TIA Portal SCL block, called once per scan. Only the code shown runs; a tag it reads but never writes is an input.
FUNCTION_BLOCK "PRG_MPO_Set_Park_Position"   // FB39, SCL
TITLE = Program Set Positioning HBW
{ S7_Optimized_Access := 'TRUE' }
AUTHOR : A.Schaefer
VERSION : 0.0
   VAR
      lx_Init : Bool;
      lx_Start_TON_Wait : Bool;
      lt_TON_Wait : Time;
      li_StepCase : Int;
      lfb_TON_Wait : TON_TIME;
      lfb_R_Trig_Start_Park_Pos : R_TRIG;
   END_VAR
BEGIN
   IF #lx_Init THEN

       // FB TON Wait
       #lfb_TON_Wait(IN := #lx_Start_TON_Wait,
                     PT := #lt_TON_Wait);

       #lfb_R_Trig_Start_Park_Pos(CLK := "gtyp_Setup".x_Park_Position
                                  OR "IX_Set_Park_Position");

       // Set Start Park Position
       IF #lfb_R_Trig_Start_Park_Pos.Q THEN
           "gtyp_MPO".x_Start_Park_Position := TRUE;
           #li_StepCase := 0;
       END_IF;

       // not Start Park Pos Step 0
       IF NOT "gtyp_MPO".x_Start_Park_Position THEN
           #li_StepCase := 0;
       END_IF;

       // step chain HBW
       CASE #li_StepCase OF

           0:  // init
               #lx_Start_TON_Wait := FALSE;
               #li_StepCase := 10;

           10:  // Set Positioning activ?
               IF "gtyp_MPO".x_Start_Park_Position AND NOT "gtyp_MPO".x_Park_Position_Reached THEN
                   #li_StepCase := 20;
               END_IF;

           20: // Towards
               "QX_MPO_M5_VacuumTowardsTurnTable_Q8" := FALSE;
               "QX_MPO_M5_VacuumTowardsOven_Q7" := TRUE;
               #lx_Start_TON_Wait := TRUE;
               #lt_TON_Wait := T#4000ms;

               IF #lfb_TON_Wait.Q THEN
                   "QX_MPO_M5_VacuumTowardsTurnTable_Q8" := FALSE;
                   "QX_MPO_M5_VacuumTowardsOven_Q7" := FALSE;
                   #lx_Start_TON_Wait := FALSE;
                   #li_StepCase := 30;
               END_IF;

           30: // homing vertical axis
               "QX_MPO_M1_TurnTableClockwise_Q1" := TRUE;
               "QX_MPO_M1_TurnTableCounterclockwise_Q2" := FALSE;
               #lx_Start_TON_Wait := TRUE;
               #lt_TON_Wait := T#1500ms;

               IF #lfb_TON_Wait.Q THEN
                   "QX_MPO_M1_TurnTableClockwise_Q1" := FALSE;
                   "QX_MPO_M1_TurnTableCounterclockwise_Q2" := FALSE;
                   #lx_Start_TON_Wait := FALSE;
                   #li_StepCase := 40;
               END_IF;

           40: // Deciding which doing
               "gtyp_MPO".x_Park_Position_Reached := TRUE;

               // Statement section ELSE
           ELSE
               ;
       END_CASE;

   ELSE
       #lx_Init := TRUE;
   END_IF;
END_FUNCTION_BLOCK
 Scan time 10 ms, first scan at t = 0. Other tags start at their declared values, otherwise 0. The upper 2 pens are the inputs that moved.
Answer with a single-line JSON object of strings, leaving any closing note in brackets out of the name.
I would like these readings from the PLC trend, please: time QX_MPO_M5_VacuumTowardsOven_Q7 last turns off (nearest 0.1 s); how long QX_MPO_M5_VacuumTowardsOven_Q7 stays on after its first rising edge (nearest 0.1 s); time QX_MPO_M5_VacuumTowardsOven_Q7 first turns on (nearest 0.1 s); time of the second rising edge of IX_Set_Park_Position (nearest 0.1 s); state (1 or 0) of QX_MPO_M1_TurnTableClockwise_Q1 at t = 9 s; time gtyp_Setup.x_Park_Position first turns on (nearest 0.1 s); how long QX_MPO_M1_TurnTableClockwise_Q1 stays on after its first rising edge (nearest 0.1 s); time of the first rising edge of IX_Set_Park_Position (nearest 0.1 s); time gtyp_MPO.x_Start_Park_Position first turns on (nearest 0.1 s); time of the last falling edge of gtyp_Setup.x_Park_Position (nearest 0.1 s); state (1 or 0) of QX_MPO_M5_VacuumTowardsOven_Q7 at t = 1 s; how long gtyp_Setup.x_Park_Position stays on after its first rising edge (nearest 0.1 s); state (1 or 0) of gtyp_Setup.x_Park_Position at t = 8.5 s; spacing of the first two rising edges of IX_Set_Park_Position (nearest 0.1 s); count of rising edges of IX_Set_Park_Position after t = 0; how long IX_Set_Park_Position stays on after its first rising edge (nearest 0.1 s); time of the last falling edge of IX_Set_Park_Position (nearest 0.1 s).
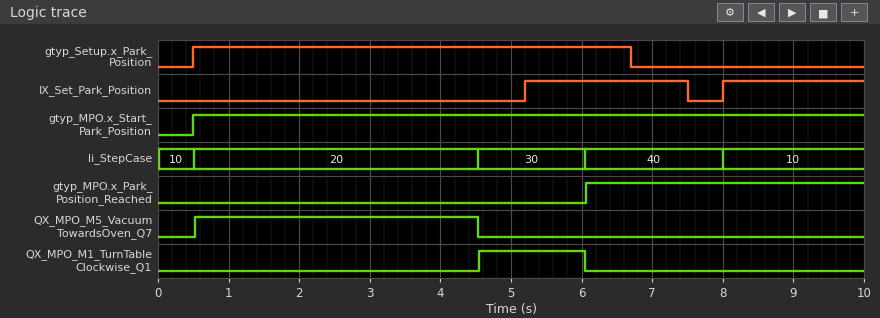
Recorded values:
{"time QX_MPO_M5_VacuumTowardsOven_Q7 last turns off": "4.5 s", "how long QX_MPO_M5_VacuumTowardsOven_Q7 stays on after its first rising edge": "4.0 s", "time QX_MPO_M5_VacuumTowardsOven_Q7 first turns on": "0.5 s", "time of the second rising edge of IX_Set_Park_Position": "8.0 s", "state (1 or 0) of QX_MPO_M1_TurnTableClockwise_Q1 at t = 9 s": "0", "time gtyp_Setup.x_Park_Position first turns on": "0.5 s", "how long QX_MPO_M1_TurnTableClockwise_Q1 stays on after its first rising edge": "1.5 s", "time of the first rising edge of IX_Set_Park_Position": "5.2 s", "time gtyp_MPO.x_Start_Park_Position first turns on": "0.5 s", "time of the last falling edge of gtyp_Setup.x_Park_Position": "6.7 s", "state (1 or 0) of QX_MPO_M5_VacuumTowardsOven_Q7 at t = 1 s": "1", "how long gtyp_Setup.x_Park_Position stays on after its first rising edge": "6.2 s", "state (1 or 0) of gtyp_Setup.x_Park_Position at t = 8.5 s": "0", "spacing of the first two rising edges of IX_Set_Park_Position": "2.8 s", "count of rising edges of IX_Set_Park_Position after t = 0": "2", "how long IX_Set_Park_Position stays on after its first rising edge": "2.3 s", "time of the last falling edge of IX_Set_Park_Position": "7.5 s"}
